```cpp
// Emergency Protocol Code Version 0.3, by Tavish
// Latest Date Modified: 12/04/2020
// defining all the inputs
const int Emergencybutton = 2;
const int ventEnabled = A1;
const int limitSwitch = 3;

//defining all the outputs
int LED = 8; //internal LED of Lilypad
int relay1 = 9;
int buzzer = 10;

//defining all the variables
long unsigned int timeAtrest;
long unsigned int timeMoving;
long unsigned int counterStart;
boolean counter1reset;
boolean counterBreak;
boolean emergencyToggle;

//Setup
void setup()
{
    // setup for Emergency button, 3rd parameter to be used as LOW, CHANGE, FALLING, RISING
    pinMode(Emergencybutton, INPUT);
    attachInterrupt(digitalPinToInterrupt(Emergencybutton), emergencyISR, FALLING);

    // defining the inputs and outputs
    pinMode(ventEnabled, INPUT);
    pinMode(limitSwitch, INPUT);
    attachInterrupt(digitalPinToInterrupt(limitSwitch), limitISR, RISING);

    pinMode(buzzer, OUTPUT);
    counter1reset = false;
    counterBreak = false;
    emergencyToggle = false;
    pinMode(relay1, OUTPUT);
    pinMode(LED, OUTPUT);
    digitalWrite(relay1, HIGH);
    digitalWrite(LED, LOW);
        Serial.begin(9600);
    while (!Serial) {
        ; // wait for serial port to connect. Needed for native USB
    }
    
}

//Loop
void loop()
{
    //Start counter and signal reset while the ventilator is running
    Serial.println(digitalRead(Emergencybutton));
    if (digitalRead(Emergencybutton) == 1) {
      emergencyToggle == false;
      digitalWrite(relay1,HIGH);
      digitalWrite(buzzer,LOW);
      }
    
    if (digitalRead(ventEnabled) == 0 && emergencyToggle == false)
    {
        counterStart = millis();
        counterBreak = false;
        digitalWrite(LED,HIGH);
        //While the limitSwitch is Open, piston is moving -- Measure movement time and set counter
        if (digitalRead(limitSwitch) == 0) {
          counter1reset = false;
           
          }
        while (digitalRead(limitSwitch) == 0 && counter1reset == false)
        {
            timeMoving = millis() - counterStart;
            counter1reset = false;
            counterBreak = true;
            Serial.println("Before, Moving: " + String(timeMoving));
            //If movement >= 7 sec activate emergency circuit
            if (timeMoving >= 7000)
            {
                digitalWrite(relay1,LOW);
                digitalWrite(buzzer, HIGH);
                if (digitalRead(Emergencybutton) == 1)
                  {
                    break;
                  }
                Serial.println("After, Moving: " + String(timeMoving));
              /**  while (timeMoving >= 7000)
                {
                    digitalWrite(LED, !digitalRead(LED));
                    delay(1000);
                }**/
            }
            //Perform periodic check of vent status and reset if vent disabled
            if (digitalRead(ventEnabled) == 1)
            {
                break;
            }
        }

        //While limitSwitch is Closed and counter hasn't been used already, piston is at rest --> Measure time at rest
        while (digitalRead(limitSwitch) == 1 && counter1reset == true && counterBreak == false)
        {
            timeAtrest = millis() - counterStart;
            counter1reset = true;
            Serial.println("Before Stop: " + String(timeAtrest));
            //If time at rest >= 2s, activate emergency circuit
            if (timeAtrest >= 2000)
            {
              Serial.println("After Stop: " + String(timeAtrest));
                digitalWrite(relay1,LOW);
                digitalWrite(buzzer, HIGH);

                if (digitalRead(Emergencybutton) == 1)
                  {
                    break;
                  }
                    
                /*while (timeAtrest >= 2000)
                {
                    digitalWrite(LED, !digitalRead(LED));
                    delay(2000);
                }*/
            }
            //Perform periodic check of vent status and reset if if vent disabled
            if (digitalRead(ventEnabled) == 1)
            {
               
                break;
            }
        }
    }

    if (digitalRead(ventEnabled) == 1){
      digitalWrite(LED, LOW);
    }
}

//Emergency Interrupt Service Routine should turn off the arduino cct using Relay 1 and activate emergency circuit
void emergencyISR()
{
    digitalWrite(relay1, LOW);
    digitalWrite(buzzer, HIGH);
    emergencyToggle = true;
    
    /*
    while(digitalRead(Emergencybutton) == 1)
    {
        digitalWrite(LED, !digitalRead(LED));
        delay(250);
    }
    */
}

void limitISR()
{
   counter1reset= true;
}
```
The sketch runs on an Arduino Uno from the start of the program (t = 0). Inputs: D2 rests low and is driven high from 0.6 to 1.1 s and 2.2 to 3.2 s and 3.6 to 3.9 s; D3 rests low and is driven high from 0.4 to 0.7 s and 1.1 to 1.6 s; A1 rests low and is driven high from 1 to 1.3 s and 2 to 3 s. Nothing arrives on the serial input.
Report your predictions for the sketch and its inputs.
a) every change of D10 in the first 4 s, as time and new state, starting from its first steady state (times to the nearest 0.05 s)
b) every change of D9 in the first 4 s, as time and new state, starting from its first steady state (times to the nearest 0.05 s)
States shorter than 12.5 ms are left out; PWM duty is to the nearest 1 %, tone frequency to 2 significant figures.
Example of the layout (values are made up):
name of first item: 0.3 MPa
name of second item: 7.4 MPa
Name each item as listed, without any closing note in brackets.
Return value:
every change of D10 in the first 4 s, as time and new state, starting from its first steady state: 0 s low; 1.1 s high; 2.2 s low; 3.2 s high; 3.6 s low; 3.9 s high
every change of D9 in the first 4 s, as time and new state, starting from its first steady state: 0 s high; 1.1 s low; 2.2 s high; 3.2 s low; 3.6 s high; 3.9 s low
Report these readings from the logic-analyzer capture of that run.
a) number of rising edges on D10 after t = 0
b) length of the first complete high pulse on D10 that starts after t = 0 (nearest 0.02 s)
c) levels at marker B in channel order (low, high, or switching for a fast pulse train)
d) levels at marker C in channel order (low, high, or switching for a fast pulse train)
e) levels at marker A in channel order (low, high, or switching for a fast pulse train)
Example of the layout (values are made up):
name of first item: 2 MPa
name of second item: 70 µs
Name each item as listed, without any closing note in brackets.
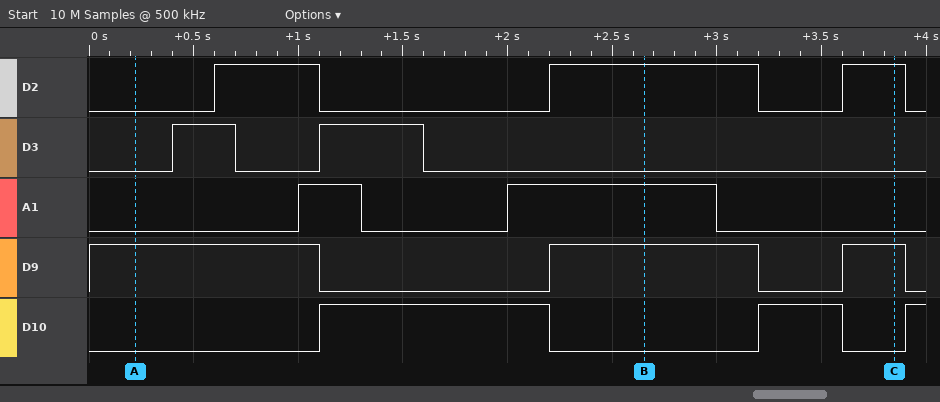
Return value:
number of rising edges on D10 after t = 0: 3
length of the first complete high pulse on D10 that starts after t = 0: 1.10 s
levels at marker B in channel order: D2 high, D3 low, A1 high, D9 high, D10 low
levels at marker C in channel order: D2 high, D3 low, A1 low, D9 high, D10 low
levels at marker A in channel order: D2 low, D3 low, A1 low, D9 high, D10 low
